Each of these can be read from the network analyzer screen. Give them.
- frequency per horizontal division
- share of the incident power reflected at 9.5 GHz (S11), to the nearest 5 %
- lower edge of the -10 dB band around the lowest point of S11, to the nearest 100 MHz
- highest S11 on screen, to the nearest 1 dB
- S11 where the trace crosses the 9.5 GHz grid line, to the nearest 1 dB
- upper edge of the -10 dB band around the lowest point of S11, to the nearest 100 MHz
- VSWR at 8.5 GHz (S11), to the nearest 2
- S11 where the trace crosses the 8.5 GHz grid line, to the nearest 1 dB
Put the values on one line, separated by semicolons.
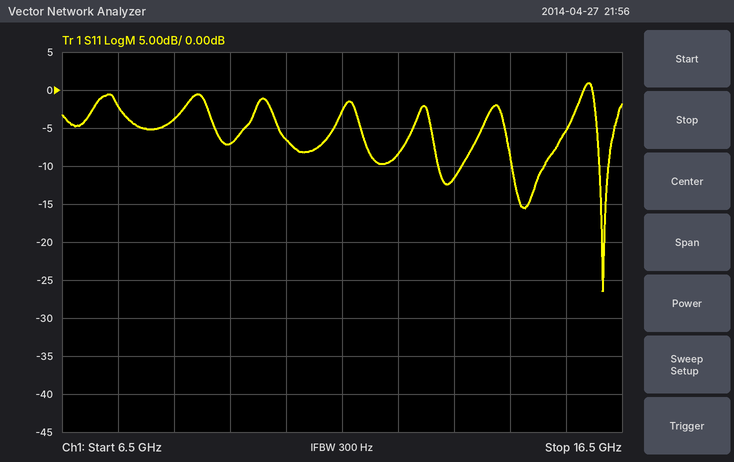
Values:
1 GHz; 20 %; 16.1 GHz; 1 dB; -7 dB; 16.3 GHz; 4; -4 dB
